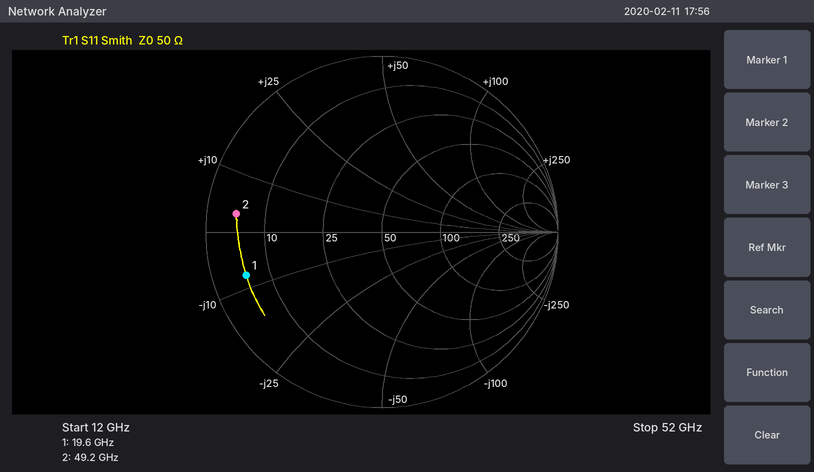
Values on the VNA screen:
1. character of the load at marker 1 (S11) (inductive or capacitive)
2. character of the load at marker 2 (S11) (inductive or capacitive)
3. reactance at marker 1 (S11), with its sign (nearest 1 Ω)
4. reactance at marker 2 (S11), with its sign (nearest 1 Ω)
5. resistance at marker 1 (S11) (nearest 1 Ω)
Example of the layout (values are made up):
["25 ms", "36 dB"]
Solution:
["capacitive", "inductive", "-8 Ω", "+3 Ω", "5 Ω"]
